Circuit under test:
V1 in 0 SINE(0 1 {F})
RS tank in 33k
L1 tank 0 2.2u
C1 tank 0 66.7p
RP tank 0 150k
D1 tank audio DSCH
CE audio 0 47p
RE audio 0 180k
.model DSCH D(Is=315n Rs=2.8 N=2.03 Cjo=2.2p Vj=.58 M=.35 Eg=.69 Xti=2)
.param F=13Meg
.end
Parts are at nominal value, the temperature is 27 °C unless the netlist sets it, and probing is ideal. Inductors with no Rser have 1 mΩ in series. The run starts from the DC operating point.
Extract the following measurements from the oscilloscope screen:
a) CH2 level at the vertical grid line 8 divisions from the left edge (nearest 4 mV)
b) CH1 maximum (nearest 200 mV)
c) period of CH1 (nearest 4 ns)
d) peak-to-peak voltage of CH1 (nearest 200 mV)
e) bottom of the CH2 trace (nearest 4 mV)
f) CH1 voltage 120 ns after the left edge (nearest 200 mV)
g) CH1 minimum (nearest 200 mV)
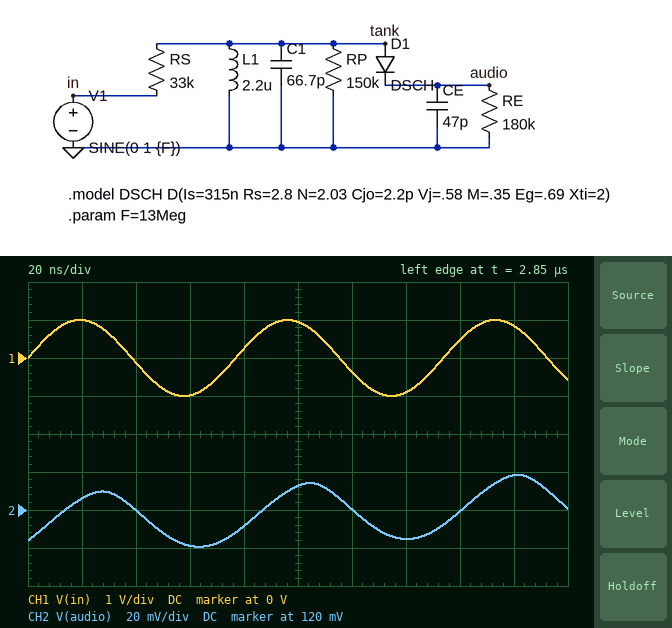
120 mV
1.0 V
76 ns
2.0 V
100 mV
-400 mV
-1.0 V
